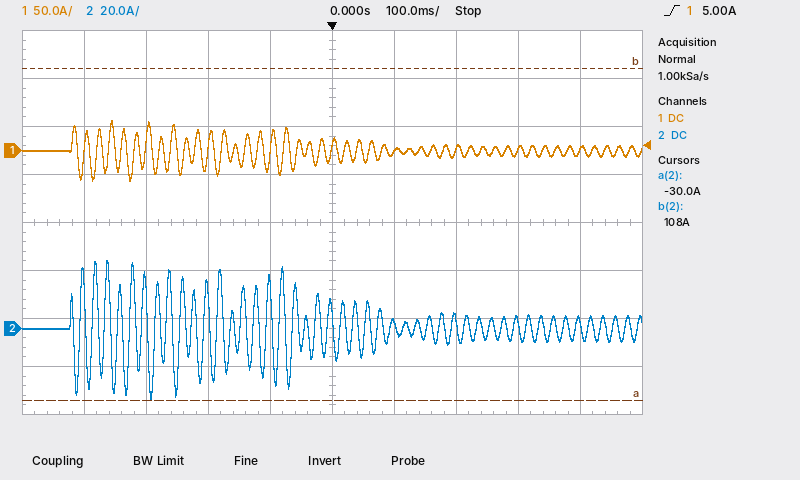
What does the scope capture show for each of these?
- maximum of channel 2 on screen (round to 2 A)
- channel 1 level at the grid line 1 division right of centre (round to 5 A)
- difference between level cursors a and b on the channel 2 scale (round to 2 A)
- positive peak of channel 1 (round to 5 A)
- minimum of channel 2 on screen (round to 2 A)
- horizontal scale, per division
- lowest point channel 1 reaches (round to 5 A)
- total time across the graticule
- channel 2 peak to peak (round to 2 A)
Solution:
28 A
0 A
138 A
30 A
-30 A
100 ms
-30 A
1 s
58 A
